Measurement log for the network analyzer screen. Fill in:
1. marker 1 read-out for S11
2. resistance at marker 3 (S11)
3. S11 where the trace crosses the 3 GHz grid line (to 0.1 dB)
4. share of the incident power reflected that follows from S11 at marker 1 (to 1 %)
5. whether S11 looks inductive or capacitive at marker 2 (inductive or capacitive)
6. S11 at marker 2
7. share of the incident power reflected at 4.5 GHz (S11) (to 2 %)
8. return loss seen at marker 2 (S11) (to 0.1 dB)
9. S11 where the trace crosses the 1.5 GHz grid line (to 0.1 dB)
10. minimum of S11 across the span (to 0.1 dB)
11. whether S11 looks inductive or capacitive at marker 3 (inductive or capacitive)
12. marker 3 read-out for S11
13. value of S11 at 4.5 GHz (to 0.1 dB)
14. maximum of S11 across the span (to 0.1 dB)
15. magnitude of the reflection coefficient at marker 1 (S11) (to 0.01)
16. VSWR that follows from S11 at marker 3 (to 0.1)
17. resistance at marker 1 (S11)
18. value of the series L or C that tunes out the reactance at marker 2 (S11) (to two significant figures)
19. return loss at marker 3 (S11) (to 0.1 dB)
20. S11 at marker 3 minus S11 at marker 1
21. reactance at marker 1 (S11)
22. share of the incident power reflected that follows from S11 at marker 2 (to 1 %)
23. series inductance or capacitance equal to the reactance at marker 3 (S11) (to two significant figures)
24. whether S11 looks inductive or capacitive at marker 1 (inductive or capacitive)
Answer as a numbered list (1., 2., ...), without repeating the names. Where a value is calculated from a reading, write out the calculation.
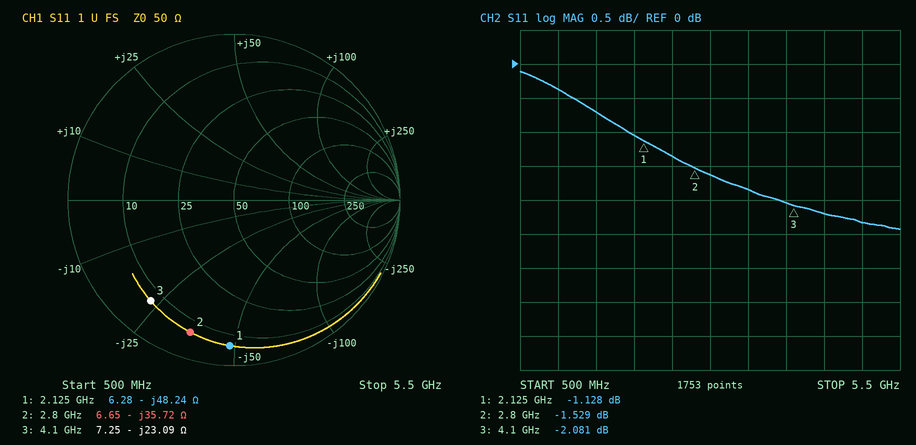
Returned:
1. -1.128 dB
2. 7.25 Ω
3. -1.6 dB
4. 10^(-1.128/10) ≈ 77 %
5. capacitive
6. -1.529 dB
7. 10^(-2.2/10) ≈ 60 %
8. 1.5 dB
9. -0.7 dB
10. -2.4 dB
11. capacitive
12. -2.081 dB
13. -2.2 dB
14. -0.1 dB
15. 0.88
16. (1 + 0.7870)/(1 − 0.7870) ≈ 8.4
17. 6.28 Ω
18. L = 35.72 Ω/(2π × 2.8 GHz) ≈ 2.0 nH
19. 2.1 dB
20. -2.081 − (-1.128) = -0.953 dB
21. -48.24 Ω
22. 10^(-1.529/10) ≈ 70 %
23. C = 1/(2π × 4.1 GHz × 23.09 Ω) ≈ 1.7 pF
24. capacitive
